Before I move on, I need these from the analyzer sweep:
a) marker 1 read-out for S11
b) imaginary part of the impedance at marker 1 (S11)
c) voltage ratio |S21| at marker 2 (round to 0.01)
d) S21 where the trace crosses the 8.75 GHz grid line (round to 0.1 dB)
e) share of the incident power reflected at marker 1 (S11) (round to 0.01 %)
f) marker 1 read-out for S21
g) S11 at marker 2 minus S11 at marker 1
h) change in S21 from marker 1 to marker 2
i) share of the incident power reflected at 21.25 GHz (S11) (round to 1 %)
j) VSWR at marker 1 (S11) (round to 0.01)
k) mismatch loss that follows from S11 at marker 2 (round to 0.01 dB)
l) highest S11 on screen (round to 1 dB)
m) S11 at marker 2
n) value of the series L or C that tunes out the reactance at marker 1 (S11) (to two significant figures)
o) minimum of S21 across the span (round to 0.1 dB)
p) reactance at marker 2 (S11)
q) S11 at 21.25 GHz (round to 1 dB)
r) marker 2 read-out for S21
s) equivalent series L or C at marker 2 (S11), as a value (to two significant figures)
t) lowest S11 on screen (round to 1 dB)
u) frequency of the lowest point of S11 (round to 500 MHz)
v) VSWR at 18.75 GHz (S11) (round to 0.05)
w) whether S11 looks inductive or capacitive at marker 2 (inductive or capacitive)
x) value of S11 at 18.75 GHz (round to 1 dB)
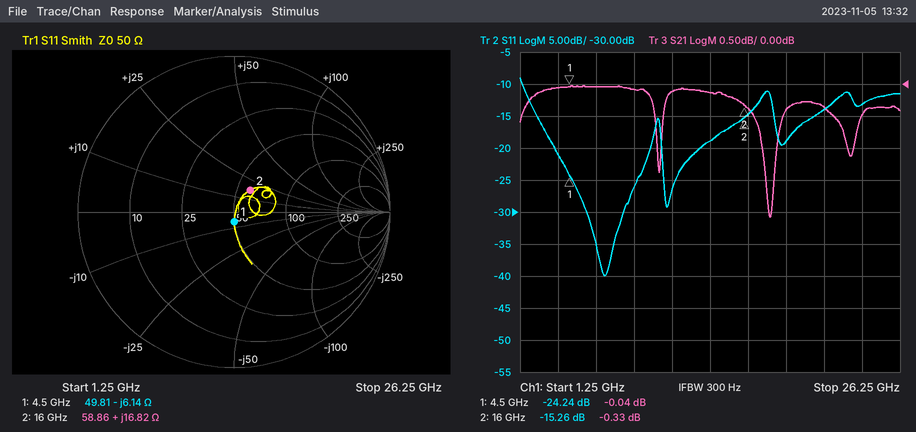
-24.24 dB
-6.14 Ω
0.96
-0.1 dB
0.38 %
-0.04 dB
8.98 dB
-0.29 dB
4 %
1.13
0.13 dB
-9 dB
-15.26 dB
220 pH
-2.1 dB
+16.82 Ω
-14 dB
-0.33 dB
170 pH
-40 dB
7.0 GHz
1.25
inductive
-19 dB
